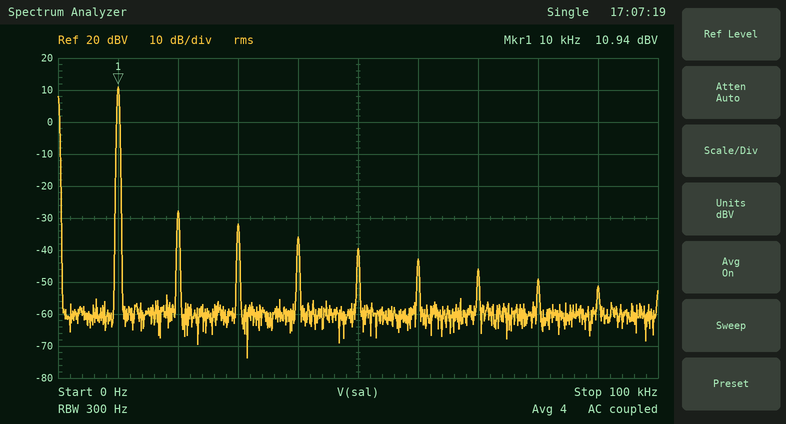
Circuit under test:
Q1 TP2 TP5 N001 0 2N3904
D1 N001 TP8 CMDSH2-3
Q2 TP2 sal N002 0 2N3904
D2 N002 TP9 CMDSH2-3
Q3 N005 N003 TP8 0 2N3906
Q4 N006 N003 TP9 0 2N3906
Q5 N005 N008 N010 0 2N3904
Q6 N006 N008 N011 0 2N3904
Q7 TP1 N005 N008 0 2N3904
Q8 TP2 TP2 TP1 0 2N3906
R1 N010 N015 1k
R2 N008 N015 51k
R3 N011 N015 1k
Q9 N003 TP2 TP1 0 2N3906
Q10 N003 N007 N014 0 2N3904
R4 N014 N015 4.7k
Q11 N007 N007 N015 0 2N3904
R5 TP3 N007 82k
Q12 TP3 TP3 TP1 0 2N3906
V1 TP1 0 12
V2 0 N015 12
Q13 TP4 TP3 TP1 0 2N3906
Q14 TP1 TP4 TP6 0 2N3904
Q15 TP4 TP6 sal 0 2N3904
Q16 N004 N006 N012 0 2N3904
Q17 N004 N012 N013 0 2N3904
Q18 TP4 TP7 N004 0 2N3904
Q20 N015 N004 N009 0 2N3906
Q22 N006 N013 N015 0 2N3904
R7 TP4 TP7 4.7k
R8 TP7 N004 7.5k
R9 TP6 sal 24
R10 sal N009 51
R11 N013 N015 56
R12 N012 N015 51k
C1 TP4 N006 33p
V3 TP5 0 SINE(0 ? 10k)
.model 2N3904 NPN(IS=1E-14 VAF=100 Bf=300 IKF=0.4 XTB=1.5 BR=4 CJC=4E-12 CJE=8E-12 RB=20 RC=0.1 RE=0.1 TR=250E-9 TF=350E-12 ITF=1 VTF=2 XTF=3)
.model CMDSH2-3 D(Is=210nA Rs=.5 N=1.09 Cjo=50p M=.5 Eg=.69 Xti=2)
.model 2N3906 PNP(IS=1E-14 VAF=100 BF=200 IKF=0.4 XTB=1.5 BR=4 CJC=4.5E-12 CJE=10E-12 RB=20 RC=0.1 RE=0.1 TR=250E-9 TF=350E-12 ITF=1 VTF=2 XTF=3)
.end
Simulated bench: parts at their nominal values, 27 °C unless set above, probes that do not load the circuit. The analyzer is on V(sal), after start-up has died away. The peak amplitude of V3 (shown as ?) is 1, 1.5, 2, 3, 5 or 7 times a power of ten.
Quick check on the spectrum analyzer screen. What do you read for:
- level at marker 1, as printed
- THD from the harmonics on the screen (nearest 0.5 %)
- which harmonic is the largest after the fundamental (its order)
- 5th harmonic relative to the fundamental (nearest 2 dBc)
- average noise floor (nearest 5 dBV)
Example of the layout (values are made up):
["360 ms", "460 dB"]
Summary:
["10.94 dBV", "1.5 %", "2", "-50 dBc", "-60 dBV"]
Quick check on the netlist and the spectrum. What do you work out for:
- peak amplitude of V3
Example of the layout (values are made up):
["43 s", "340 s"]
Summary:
["5 V"]
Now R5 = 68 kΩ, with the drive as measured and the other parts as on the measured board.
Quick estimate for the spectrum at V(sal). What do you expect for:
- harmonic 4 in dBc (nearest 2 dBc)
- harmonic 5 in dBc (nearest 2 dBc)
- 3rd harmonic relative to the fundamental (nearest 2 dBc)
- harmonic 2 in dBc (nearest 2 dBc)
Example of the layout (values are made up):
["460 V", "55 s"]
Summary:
["-52 dBc", "-56 dBc", "-48 dBc", "-42 dBc"]
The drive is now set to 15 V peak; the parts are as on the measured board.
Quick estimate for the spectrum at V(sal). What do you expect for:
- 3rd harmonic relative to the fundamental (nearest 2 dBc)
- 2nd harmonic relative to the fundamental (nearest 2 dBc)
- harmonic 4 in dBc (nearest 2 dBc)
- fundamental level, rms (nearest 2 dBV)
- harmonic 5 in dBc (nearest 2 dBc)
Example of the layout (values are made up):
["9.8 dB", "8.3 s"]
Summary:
["10 dBc", "14 dBc", "-10 dBc", "-2 dBV", "0 dBc"]
